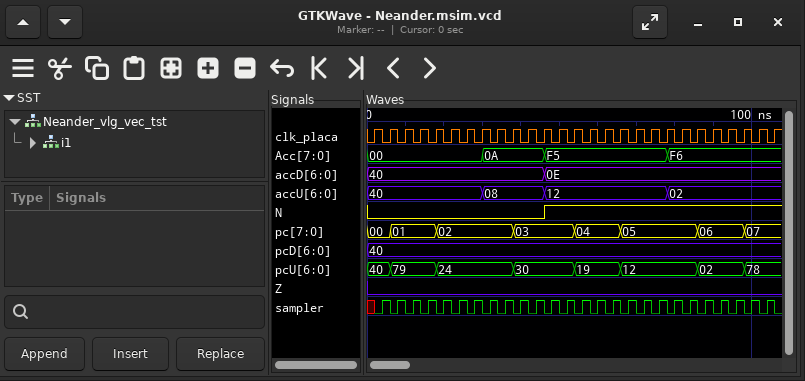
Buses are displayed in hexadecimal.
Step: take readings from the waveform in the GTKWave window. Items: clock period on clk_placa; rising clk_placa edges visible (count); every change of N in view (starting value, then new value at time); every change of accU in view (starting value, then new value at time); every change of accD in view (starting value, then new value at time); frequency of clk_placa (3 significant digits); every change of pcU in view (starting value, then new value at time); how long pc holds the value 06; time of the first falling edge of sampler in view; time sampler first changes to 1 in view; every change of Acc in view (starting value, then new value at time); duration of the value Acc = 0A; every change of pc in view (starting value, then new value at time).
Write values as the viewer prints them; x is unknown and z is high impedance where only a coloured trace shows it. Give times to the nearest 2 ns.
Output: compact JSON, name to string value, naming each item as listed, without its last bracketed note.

{"clock period on clk_placa": "4 ns", "rising clk_placa edges visible": "27", "every change of N in view": "0, 1 at 46 ns", "every change of accU in view": "40, 08 at 30 ns, 12 at 46 ns, 02 at 78 ns", "every change of accD in view": "40, 0E at 46 ns", "frequency of clk_placa": "250 MHz", "every change of pcU in view": "40, 79 at 6 ns, 24 at 18 ns, 30 at 38 ns, 19 at 54 ns, 12 at 66 ns, 02 at 86 ns, 78 at 98 ns", "how long pc holds the value 06": "12 ns", "time of the first falling edge of sampler in view": "6 ns", "time sampler first changes to 1 in view": "4 ns", "every change of Acc in view": "00, 0A at 30 ns, F5 at 46 ns, F6 at 78 ns", "duration of the value Acc = 0A": "16 ns", "every change of pc in view": "00, 01 at 6 ns, 02 at 18 ns, 03 at 38 ns, 04 at 54 ns, 05 at 66 ns, 06 at 86 ns, 07 at 98 ns"}
